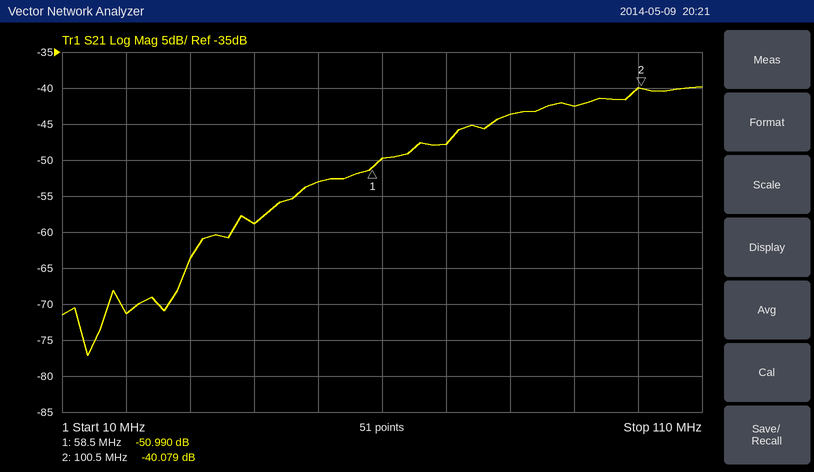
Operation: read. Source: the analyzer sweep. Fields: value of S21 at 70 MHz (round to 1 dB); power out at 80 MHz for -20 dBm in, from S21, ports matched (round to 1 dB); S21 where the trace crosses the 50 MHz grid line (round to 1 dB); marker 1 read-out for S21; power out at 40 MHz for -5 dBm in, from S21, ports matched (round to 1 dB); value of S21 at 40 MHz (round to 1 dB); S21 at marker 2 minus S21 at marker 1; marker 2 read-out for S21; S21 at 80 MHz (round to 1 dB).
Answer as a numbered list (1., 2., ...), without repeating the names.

1. -48 dB
2. -64 dBm
3. -53 dB
4. -50.990 dB
5. -64 dBm
6. -59 dB
7. 10.911 dB
8. -40.079 dB
9. -44 dB
